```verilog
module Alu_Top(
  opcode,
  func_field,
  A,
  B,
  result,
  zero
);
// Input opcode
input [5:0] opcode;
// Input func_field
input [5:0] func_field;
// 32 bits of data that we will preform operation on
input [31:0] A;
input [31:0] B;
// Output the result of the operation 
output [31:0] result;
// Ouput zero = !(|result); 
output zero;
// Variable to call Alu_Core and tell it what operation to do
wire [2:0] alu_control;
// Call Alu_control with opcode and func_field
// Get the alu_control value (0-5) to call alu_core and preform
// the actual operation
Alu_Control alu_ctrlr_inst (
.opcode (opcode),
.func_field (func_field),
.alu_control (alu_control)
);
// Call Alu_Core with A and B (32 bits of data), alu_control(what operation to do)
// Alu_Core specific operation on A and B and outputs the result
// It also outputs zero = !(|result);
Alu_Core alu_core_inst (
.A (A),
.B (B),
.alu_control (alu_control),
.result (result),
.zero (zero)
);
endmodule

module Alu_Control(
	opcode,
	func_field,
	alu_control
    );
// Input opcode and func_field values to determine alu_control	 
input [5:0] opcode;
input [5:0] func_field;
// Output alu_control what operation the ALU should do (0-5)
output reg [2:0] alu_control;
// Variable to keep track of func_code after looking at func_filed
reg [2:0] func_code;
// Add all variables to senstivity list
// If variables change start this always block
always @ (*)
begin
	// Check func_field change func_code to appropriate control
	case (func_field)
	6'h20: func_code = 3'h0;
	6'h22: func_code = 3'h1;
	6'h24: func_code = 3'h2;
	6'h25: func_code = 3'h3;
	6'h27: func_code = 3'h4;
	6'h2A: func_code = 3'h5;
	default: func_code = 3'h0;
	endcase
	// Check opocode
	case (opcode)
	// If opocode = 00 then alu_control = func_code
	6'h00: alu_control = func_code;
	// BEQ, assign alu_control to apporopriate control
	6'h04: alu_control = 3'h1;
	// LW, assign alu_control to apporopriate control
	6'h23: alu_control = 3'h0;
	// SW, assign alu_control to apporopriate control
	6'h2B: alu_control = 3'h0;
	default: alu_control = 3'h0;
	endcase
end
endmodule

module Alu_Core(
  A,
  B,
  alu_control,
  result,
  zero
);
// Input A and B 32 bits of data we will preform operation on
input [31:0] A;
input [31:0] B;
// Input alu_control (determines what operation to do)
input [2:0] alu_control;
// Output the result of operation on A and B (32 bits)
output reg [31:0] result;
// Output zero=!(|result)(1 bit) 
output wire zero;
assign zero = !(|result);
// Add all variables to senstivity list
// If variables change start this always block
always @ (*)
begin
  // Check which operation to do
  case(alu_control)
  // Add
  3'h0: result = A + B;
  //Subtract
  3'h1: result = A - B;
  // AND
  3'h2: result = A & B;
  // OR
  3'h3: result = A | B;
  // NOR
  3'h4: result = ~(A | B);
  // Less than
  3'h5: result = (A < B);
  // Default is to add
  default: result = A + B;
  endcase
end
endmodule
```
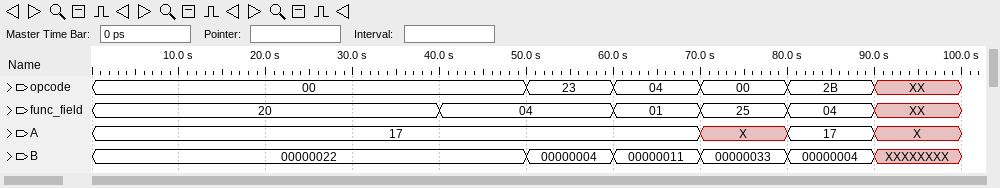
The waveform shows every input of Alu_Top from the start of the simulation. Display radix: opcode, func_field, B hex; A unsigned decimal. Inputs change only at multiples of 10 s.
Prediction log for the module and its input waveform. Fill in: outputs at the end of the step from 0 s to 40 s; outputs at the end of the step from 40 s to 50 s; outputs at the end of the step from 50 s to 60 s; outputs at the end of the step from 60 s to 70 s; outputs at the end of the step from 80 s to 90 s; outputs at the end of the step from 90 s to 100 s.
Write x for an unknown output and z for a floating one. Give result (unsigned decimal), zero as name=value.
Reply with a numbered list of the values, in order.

1. result=51, zero=0
2. result=51, zero=0
3. result=21, zero=0
4. result=0, zero=1
5. result=21, zero=0
6. result=x, zero=x
